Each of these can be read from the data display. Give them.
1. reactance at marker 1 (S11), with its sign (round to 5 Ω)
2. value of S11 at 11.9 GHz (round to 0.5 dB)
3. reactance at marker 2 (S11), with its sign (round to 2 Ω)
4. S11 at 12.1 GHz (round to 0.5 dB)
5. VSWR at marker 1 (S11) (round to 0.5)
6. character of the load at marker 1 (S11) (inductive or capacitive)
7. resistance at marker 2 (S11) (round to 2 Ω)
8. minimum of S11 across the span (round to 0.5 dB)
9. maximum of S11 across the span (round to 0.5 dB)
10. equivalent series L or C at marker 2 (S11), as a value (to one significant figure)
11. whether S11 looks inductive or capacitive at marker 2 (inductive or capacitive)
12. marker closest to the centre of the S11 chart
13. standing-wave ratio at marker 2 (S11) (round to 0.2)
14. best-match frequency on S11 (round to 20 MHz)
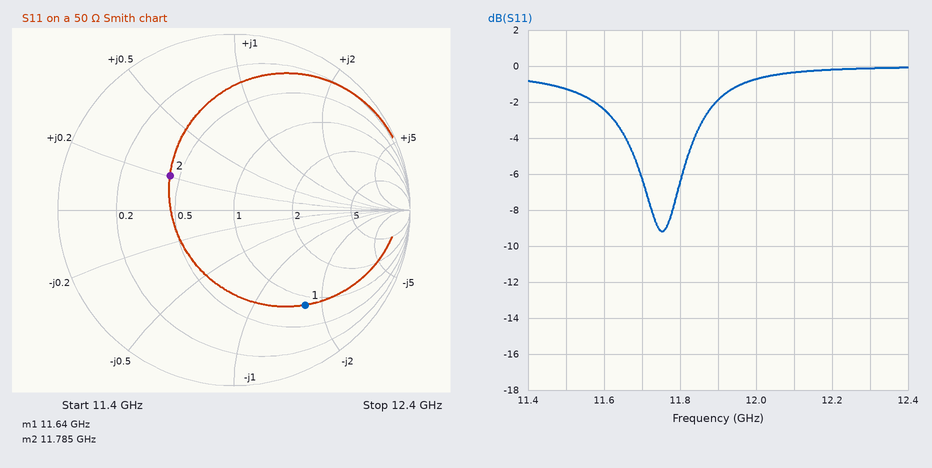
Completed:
-85 Ω
-2.0 dB
+10 Ω
-0.5 dB
5.0
capacitive
22 Ω
-9.0 dB
0.0 dB
100 pH
inductive
marker 2
2.4
11.76 GHz
